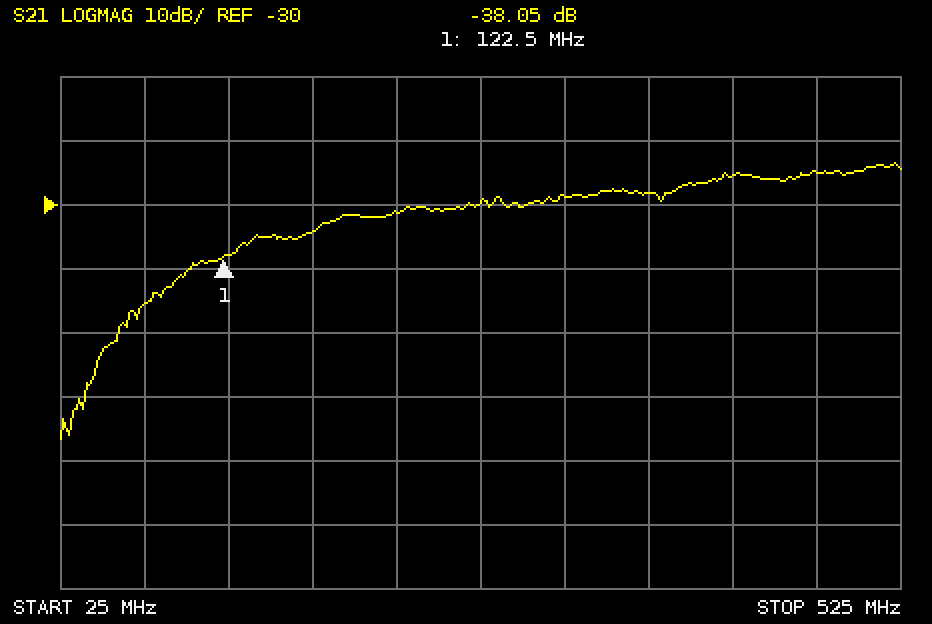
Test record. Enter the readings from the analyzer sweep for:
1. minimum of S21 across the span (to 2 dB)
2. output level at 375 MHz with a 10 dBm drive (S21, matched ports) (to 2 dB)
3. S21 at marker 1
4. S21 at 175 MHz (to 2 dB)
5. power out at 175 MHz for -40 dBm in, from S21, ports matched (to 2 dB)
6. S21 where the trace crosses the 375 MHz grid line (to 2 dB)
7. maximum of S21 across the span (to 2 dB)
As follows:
-66 dB
-18 dBm
-38.05 dB
-34 dB
-74 dBm
-28 dB
-24 dB
